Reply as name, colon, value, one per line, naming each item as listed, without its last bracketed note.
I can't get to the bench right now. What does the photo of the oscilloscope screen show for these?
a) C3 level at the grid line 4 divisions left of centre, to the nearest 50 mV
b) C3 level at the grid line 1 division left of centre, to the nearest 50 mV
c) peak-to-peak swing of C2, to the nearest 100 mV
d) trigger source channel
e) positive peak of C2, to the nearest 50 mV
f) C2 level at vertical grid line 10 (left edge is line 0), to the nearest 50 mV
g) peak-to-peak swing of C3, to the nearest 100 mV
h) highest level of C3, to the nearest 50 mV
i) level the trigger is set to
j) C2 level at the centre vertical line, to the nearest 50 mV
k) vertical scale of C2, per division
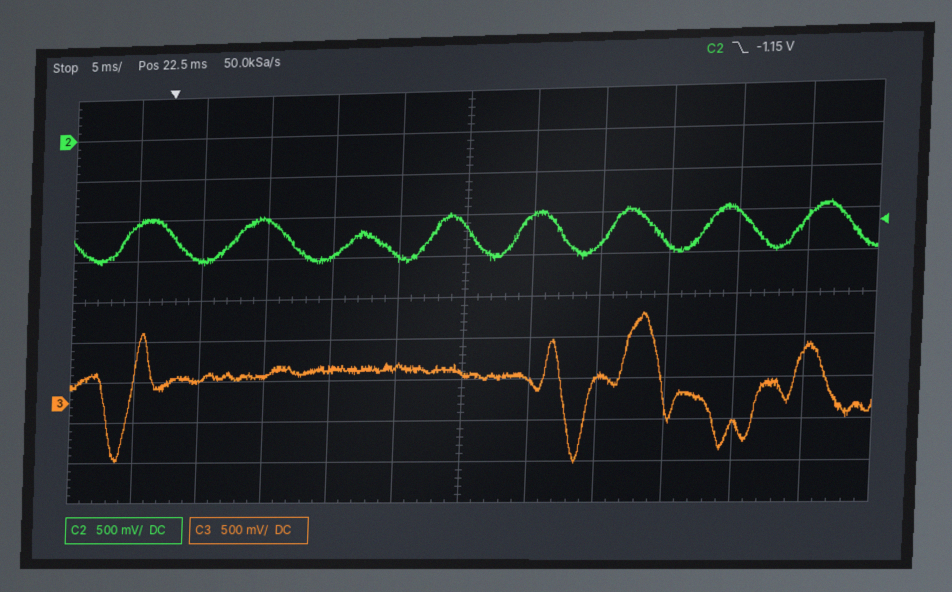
C3 level at the grid line 4 divisions left of centre, to the nearest 50 mV: 250 mV
C3 level at the grid line 1 division left of centre, to the nearest 50 mV: 400 mV
peak-to-peak swing of C2, to the nearest 100 mV: 700 mV
trigger source channel: C2
positive peak of C2, to the nearest 50 mV: -900 mV
C2 level at vertical grid line 10 (left edge is line 0), to the nearest 50 mV: -1.00 V
peak-to-peak swing of C3, to the nearest 100 mV: 1.80 V
highest level of C3, to the nearest 50 mV: 1.05 V
level the trigger is set to: -1.15 V
C2 level at the centre vertical line, to the nearest 50 mV: -1.15 V
vertical scale of C2, per division: 500 mV
